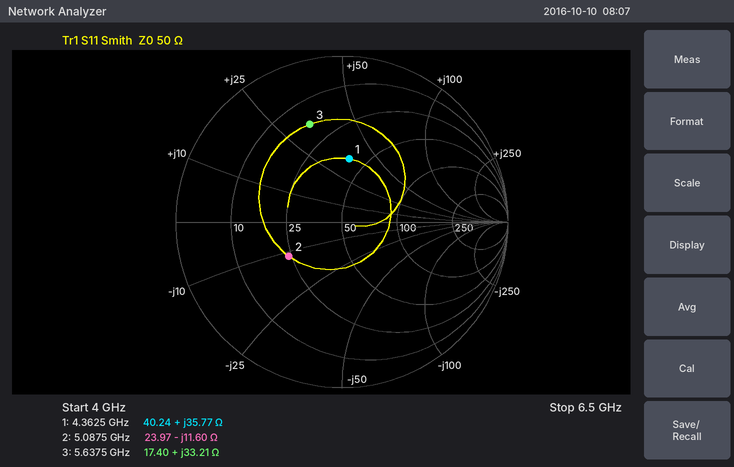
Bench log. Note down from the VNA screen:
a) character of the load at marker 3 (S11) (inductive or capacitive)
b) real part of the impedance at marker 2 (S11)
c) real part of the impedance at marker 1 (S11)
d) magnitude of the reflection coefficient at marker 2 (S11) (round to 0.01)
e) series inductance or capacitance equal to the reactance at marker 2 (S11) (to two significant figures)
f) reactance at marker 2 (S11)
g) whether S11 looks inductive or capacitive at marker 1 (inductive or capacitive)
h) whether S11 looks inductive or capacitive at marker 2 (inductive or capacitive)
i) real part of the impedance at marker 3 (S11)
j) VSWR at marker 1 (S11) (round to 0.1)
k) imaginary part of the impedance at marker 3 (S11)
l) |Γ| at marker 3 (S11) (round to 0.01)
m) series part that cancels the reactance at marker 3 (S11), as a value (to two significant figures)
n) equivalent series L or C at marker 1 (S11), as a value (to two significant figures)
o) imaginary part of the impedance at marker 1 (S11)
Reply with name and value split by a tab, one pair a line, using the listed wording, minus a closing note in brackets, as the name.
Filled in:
character of the load at marker 3 (S11)	inductive
real part of the impedance at marker 2	23.97 Ω
real part of the impedance at marker 1	40.24 Ω
magnitude of the reflection coefficient at marker 2 (S11)	0.38
series inductance or capacitance equal to the reactance at marker 2 (S11)	2.7 pF
reactance at marker 2	-11.60 Ω
whether S11 looks inductive or capacitive at marker 1	inductive
whether S11 looks inductive or capacitive at marker 2	capacitive
real part of the impedance at marker 3	17.40 Ω
VSWR at marker 1 (S11)	2.2
imaginary part of the impedance at marker 3	+33.21 Ω
|Γ| at marker 3 (S11)	0.62
series part that cancels the reactance at marker 3 (S11), as a value	850 fF
equivalent series L or C at marker 1 (S11), as a value	1.3 nH
imaginary part of the impedance at marker 1	+35.77 Ω
